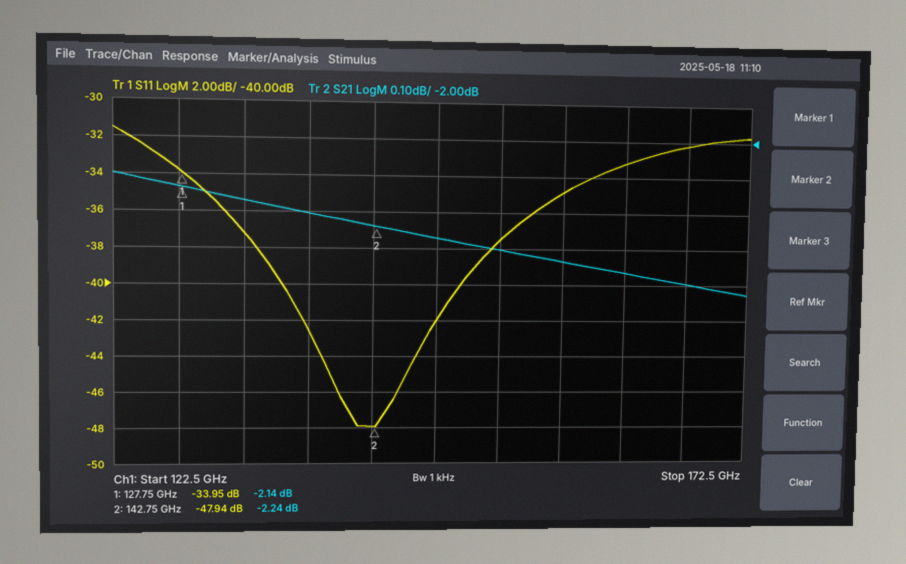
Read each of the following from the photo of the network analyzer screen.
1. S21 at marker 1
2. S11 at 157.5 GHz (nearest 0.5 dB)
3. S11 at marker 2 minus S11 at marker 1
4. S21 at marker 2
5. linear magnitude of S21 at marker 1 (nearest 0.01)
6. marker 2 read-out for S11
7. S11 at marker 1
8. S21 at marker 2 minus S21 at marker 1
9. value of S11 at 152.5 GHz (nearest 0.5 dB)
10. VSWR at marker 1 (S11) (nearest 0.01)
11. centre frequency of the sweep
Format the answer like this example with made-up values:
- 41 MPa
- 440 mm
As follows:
- -2.14 dB
- -35.0 dB
- -13.99 dB
- -2.24 dB
- 0.78
- -47.94 dB
- -33.95 dB
- -0.10 dB
- -37.5 dB
- 1.04
- 147.5 GHz
